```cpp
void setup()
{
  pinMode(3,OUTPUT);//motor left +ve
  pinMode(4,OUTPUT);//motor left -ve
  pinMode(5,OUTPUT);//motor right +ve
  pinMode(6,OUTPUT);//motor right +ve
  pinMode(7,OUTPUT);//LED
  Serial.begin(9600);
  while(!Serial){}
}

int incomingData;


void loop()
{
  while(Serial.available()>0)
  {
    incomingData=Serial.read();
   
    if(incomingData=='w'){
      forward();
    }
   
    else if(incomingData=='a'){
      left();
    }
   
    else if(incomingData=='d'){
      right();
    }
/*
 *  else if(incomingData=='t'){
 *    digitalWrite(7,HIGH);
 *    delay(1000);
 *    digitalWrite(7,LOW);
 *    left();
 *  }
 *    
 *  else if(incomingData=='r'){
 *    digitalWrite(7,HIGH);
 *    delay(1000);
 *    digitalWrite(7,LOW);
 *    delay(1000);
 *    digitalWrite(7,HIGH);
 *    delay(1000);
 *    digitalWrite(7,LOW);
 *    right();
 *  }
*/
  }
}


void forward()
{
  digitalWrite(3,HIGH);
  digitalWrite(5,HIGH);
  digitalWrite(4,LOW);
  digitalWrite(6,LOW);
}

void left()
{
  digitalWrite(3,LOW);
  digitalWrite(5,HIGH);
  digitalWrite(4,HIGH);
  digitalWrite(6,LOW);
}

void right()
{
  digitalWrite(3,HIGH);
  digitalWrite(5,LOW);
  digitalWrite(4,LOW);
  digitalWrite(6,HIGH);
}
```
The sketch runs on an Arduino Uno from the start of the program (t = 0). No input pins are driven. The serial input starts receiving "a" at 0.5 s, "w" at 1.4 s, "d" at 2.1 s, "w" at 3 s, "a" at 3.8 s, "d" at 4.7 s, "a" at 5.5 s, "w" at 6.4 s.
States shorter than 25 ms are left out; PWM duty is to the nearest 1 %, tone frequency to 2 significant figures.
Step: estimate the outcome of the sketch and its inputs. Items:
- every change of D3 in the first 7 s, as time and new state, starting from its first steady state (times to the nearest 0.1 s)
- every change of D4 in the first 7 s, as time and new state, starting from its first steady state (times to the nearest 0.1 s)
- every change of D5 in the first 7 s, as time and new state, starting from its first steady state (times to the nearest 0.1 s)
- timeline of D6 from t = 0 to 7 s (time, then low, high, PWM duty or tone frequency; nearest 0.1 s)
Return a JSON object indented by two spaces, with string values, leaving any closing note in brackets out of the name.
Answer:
{
  "every change of D3 in the first 7 s, as time and new state, starting from its first steady state": "0 s low; 1.4 s high; 3.8 s low; 4.7 s high; 5.5 s low; 6.4 s high",
  "every change of D4 in the first 7 s, as time and new state, starting from its first steady state": "0 s low; 0.5 s high; 1.4 s low; 3.8 s high; 4.7 s low; 5.5 s high; 6.4 s low",
  "every change of D5 in the first 7 s, as time and new state, starting from its first steady state": "0 s low; 0.5 s high; 2.1 s low; 3 s high; 4.7 s low; 5.5 s high",
  "timeline of D6 from t = 0 to 7 s": "0 s low; 2.1 s high; 3 s low; 4.7 s high; 5.5 s low"
}
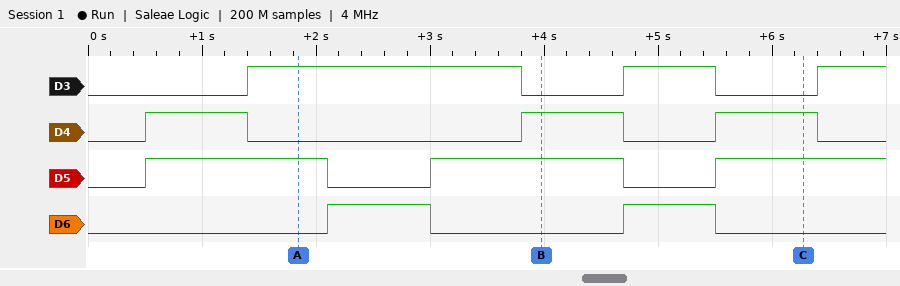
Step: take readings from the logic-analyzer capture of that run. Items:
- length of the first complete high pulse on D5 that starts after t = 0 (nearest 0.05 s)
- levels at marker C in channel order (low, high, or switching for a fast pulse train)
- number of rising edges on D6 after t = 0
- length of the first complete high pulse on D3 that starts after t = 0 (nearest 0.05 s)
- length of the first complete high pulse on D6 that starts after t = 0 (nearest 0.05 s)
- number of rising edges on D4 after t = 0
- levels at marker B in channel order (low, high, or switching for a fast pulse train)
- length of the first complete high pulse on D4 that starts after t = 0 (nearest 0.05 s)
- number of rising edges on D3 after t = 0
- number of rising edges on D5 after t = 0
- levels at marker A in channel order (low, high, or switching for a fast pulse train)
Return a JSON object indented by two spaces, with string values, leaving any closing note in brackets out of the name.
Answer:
{
  "length of the first complete high pulse on D5 that starts after t = 0": "1.60 s",
  "levels at marker C in channel order": "D3 low, D4 high, D5 high, D6 low",
  "number of rising edges on D6 after t = 0": "2",
  "length of the first complete high pulse on D3 that starts after t = 0": "2.40 s",
  "length of the first complete high pulse on D6 that starts after t = 0": "0.90 s",
  "number of rising edges on D4 after t = 0": "3",
  "levels at marker B in channel order": "D3 low, D4 high, D5 high, D6 low",
  "length of the first complete high pulse on D4 that starts after t = 0": "0.90 s",
  "number of rising edges on D3 after t = 0": "3",
  "number of rising edges on D5 after t = 0": "3",
  "levels at marker A in channel order": "D3 high, D4 low, D5 high, D6 low"
}
